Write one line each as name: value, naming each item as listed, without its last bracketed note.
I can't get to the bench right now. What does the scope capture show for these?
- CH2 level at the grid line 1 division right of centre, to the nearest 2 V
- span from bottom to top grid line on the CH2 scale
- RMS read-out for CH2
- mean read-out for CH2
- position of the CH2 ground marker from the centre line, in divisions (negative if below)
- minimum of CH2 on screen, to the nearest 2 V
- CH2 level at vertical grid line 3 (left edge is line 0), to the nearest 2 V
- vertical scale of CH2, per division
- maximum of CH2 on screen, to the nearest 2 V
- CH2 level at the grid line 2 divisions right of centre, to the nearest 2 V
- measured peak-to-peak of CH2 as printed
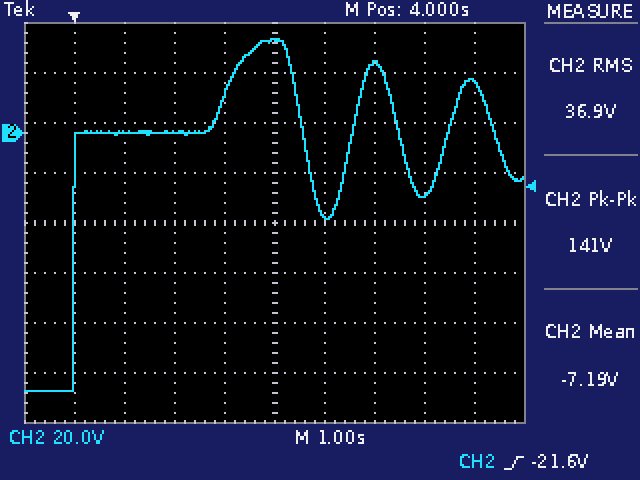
CH2 level at the grid line 1 division right of centre, to the nearest 2 V: -32 V
span from bottom to top grid line on the CH2 scale: 160 V
RMS read-out for CH2: 36.9 V
mean read-out for CH2: -7.19 V
position of the CH2 ground marker from the centre line, in divisions: +1.8 div
minimum of CH2 on screen, to the nearest 2 V: -104 V
CH2 level at vertical grid line 3 (left edge is line 0), to the nearest 2 V: 0 V
vertical scale of CH2, per division: 20 V
maximum of CH2 on screen, to the nearest 2 V: 38 V
CH2 level at the grid line 2 divisions right of centre, to the nearest 2 V: 28 V
measured peak-to-peak of CH2 as printed: 141 V
